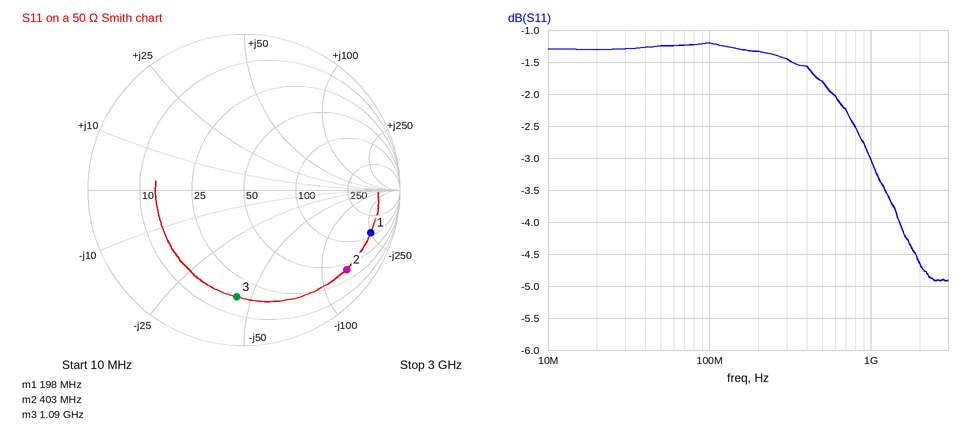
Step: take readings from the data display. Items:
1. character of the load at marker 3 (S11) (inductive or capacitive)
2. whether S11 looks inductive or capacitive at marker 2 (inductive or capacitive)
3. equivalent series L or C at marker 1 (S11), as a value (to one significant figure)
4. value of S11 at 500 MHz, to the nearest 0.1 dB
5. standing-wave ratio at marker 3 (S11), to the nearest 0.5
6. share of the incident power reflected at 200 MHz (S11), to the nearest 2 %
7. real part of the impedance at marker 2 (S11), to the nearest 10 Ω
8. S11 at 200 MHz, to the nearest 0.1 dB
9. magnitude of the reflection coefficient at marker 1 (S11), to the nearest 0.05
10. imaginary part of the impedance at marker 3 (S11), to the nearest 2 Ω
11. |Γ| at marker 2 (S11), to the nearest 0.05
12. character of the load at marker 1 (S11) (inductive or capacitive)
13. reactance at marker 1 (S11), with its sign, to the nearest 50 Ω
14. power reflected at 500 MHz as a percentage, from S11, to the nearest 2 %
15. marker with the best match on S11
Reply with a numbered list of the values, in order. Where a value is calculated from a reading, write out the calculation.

1. capacitive
2. capacitive
3. C = 1/(2π × 198 MHz × 250 Ω) ≈ 3 pF
4. -1.8 dB
5. 5.5
6. 10^(-1.3/10) ≈ 74 %
7. 40 Ω
8. -1.3 dB
9. 0.85
10. -44 Ω
11. 0.85
12. capacitive
13. -250 Ω
14. 10^(-1.8/10) ≈ 66 %
15. marker 3
